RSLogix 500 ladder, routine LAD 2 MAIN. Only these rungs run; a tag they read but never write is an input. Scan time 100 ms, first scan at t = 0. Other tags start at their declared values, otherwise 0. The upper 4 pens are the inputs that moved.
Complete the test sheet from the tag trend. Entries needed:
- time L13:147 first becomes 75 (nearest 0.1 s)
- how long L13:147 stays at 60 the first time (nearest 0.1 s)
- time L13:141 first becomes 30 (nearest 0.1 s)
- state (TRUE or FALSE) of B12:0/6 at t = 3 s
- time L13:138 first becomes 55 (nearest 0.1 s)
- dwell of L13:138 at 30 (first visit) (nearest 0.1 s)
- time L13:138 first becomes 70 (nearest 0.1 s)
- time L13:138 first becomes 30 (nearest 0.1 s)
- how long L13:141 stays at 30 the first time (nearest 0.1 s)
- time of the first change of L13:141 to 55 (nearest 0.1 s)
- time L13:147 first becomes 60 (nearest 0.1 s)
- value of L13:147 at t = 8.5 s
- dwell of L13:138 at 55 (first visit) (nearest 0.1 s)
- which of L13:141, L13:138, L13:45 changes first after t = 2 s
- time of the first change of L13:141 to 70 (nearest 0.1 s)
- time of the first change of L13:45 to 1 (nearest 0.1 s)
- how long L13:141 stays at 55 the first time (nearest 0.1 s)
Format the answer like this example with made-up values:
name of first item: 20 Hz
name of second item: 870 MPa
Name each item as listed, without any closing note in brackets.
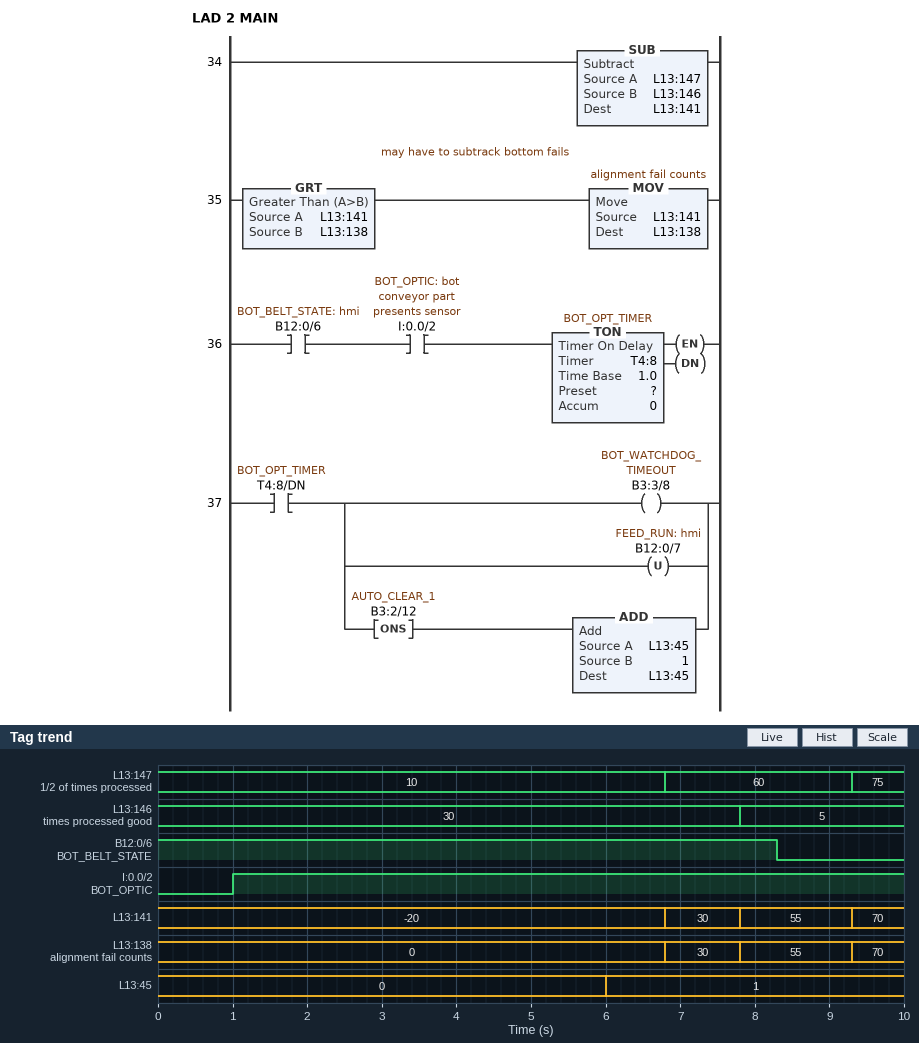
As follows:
time L13:147 first becomes 75: 9.3 s
how long L13:147 stays at 60 the first time: 2.5 s
time L13:141 first becomes 30: 6.8 s
state (TRUE or FALSE) of B12:0/6 at t = 3 s: TRUE
time L13:138 first becomes 55: 7.8 s
dwell of L13:138 at 30 (first visit): 1.0 s
time L13:138 first becomes 70: 9.3 s
time L13:138 first becomes 30: 6.8 s
how long L13:141 stays at 30 the first time: 1.0 s
time of the first change of L13:141 to 55: 7.8 s
time L13:147 first becomes 60: 6.8 s
value of L13:147 at t = 8.5 s: 60
dwell of L13:138 at 55 (first visit): 1.5 s
which of L13:141, L13:138, L13:45 changes first after t = 2 s: L13:45
time of the first change of L13:141 to 70: 9.3 s
time of the first change of L13:45 to 1: 6.0 s
how long L13:141 stays at 55 the first time: 1.5 s
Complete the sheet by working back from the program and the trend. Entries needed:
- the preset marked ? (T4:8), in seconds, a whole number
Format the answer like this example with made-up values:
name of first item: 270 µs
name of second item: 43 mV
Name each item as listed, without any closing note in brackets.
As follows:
the preset marked ? (T4:8), in seconds, a whole number: 5 s
